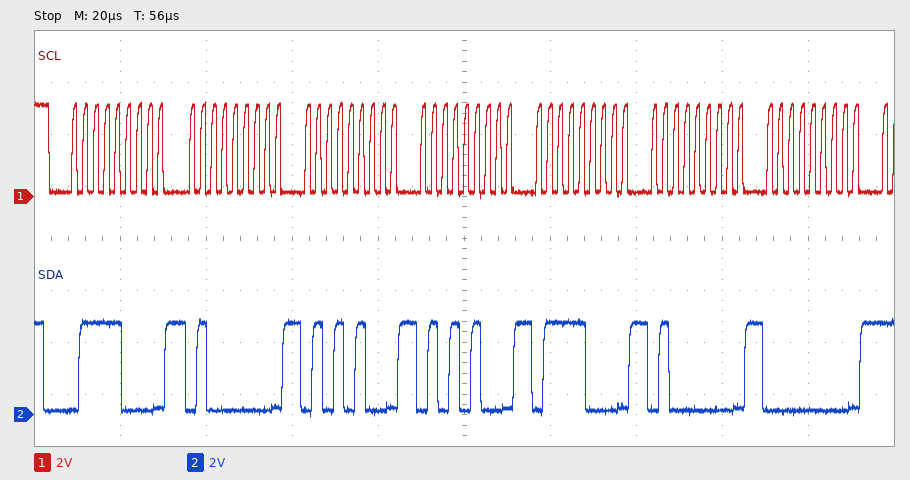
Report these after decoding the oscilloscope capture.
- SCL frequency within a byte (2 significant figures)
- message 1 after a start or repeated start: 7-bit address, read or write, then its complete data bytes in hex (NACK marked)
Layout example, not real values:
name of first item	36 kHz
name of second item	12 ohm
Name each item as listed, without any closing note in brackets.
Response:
SCL frequency within a byte	400 kHz
message 1 after a start or repeated start: 7-bit address, read or write, then its complete data bytes in hex	0x3C write: 40 54 54 78 40 00
